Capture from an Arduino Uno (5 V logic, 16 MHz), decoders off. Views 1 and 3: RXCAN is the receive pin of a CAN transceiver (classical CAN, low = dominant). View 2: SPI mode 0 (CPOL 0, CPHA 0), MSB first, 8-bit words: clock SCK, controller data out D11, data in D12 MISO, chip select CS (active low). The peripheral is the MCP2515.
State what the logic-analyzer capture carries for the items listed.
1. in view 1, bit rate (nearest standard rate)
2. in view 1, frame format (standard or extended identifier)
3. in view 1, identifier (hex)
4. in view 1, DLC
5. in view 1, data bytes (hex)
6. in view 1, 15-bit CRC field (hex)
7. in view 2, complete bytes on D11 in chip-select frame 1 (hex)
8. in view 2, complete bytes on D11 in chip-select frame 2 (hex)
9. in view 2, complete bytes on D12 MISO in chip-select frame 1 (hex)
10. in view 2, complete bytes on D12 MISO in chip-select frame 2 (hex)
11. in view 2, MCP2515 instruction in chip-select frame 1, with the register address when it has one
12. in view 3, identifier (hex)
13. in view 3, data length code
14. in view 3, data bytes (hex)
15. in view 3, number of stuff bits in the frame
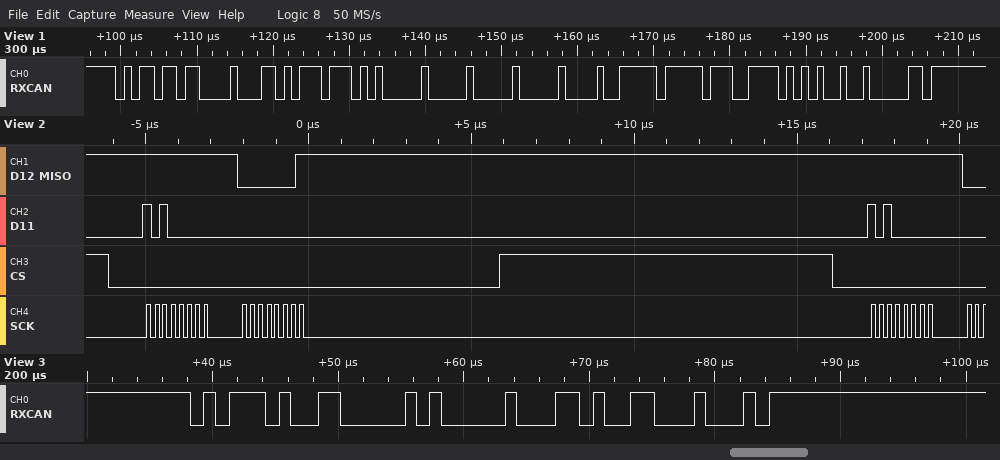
1000 kbit/s
standard
0x5B6
8
D7 75 00 00 00 9F FF 3D
0x2920
A0 00
A0
FF 01
FF
READ STATUS
0x5D3
1
00
2
